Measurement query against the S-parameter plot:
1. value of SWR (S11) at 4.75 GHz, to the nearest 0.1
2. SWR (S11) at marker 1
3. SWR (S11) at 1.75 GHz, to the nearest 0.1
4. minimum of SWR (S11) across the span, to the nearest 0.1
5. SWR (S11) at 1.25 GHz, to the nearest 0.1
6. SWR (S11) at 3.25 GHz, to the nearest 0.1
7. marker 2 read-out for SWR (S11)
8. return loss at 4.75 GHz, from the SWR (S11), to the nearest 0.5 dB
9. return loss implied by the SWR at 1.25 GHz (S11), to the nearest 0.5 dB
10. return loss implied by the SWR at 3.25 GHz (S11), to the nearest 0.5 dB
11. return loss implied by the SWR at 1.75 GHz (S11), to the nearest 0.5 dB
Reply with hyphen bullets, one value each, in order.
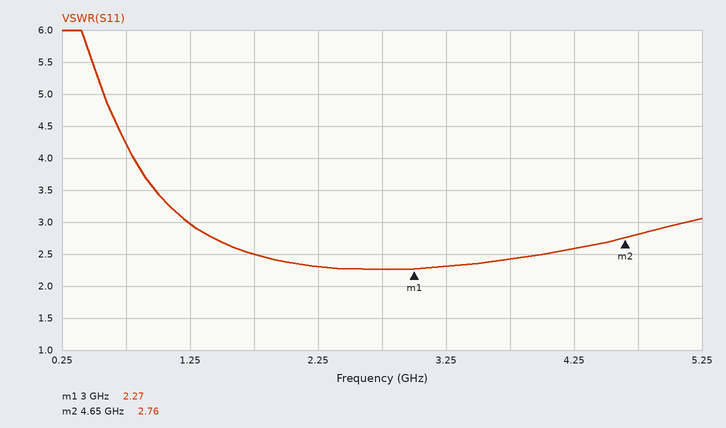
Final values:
- 2.8
- 2.27
- 2.5
- 2.3
- 3.0
- 2.3
- 2.76
- 6.5 dB
- 6.0 dB
- 8.0 dB
- 7.5 dB
